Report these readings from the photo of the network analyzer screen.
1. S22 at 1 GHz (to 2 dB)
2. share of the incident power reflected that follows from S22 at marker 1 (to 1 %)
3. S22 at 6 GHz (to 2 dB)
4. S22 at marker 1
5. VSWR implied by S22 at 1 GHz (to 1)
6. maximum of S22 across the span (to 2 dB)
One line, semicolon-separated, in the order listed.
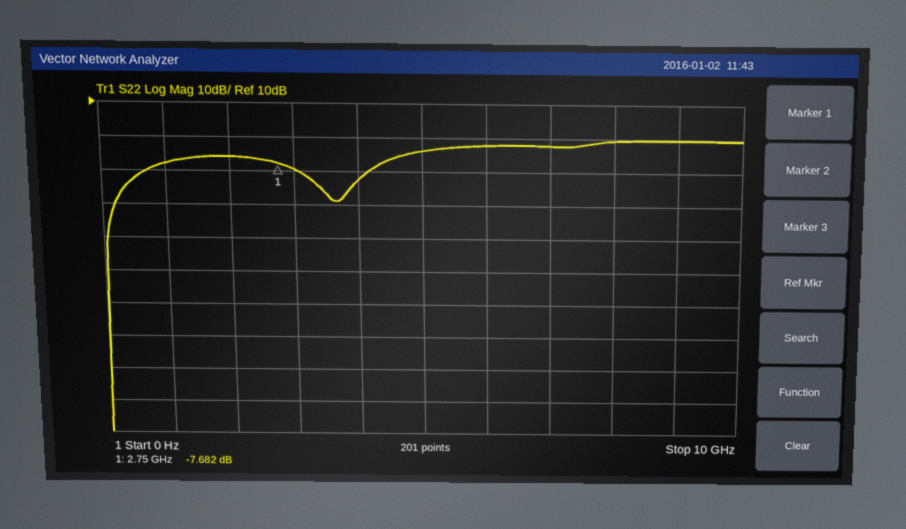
-8 dB; 17 %; -2 dB; -7.682 dB; 2; 0 dB
